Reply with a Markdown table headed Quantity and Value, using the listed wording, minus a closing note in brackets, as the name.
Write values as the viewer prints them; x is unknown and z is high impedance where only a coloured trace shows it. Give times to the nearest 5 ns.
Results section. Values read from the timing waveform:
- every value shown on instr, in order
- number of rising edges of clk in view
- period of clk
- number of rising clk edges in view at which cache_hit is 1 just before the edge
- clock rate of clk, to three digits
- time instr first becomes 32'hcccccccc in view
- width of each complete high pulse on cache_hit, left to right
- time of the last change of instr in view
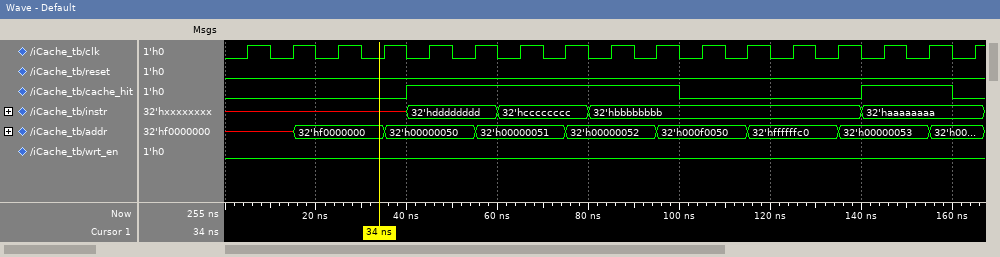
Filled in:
| Quantity | Value |
|---|---|
| every value shown on instr, in order | x, 32'hdddddddd, 32'hcccccccc, 32'hbbbbbbbb, 32'haaaaaaaa |
| number of rising edges of clk in view | 17 |
| period of clk | 10 ns |
| number of rising clk edges in view at which cache_hit is 1 just before the edge | 8 |
| clock rate of clk, to three digits | 100 MHz |
| time instr first becomes 32'hcccccccc in view | 60 ns |
| width of each complete high pulse on cache_hit, left to right | 60 ns, 20 ns |
| time of the last change of instr in view | 140 ns |
